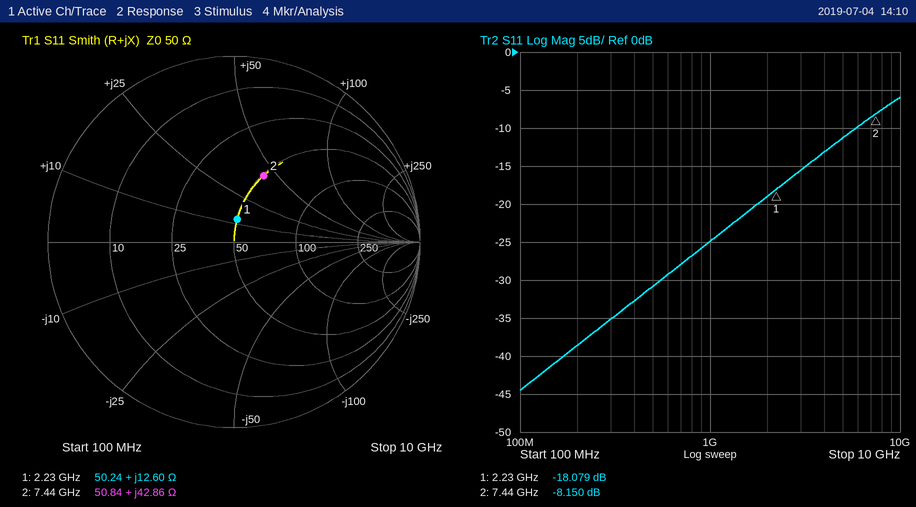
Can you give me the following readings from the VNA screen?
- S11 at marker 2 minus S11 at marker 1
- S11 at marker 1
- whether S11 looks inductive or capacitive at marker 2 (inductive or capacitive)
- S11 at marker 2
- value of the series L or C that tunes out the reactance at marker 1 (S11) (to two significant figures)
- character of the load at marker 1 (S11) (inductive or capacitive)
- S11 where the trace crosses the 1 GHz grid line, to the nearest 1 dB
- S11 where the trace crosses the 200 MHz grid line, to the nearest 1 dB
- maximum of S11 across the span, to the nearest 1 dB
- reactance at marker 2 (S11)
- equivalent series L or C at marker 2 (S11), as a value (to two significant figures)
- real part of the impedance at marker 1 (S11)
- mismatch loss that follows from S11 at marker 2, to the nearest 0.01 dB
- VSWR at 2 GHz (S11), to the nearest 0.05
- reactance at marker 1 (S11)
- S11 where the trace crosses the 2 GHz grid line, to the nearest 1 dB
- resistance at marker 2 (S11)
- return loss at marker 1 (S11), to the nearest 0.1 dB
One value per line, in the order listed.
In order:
9.929 dB
-18.079 dB
inductive
-8.150 dB
5.7 pF
inductive
-25 dB
-39 dB
-6 dB
+42.86 Ω
920 pH
50.24 Ω
0.72 dB
1.25
+12.60 Ω
-19 dB
50.84 Ω
18.1 dB
